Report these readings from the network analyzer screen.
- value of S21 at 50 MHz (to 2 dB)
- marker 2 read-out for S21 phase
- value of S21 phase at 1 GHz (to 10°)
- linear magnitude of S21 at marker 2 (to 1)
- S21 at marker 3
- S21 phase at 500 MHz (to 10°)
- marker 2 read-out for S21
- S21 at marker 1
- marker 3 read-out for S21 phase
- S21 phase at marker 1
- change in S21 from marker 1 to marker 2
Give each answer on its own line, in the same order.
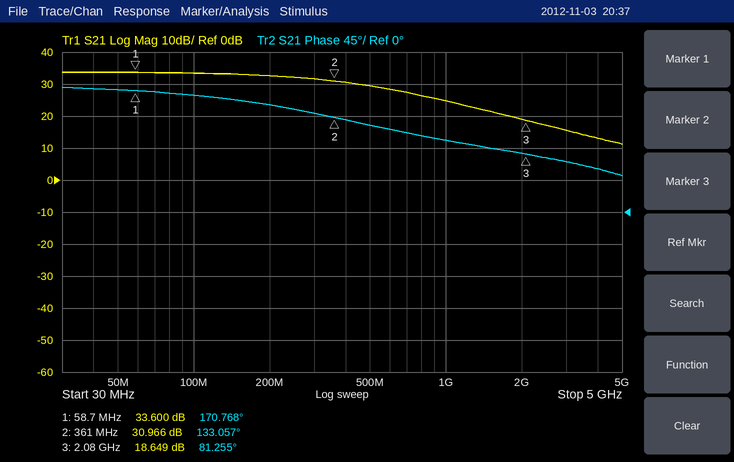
34 dB
133.057°
100°
35
18.649 dB
120°
30.966 dB
33.600 dB
81.255°
170.768°
-2.634 dB
